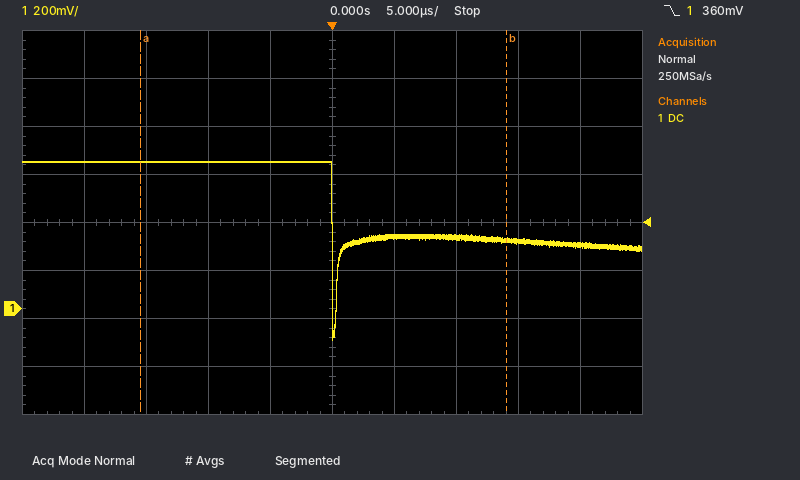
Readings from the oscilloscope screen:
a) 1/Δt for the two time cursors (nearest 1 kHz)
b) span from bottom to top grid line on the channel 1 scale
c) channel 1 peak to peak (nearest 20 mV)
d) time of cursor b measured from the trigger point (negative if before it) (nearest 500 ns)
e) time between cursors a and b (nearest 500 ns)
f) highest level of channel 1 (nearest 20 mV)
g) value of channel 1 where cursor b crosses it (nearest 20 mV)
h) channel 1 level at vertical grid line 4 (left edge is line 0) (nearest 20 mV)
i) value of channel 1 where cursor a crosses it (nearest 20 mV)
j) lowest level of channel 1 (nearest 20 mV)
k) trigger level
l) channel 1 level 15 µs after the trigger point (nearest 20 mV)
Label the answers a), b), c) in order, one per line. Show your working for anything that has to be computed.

a) 1 / 29.5 µs ≈ 34 kHz
b) 1.6 V
c) 620 mV − (-120 mV) = 740 mV
d) +14.0 µs
e) 29.5 µs
f) 620 mV
g) 280 mV
h) 620 mV
i) 620 mV
j) -120 mV
k) 360 mV
l) 280 mV
